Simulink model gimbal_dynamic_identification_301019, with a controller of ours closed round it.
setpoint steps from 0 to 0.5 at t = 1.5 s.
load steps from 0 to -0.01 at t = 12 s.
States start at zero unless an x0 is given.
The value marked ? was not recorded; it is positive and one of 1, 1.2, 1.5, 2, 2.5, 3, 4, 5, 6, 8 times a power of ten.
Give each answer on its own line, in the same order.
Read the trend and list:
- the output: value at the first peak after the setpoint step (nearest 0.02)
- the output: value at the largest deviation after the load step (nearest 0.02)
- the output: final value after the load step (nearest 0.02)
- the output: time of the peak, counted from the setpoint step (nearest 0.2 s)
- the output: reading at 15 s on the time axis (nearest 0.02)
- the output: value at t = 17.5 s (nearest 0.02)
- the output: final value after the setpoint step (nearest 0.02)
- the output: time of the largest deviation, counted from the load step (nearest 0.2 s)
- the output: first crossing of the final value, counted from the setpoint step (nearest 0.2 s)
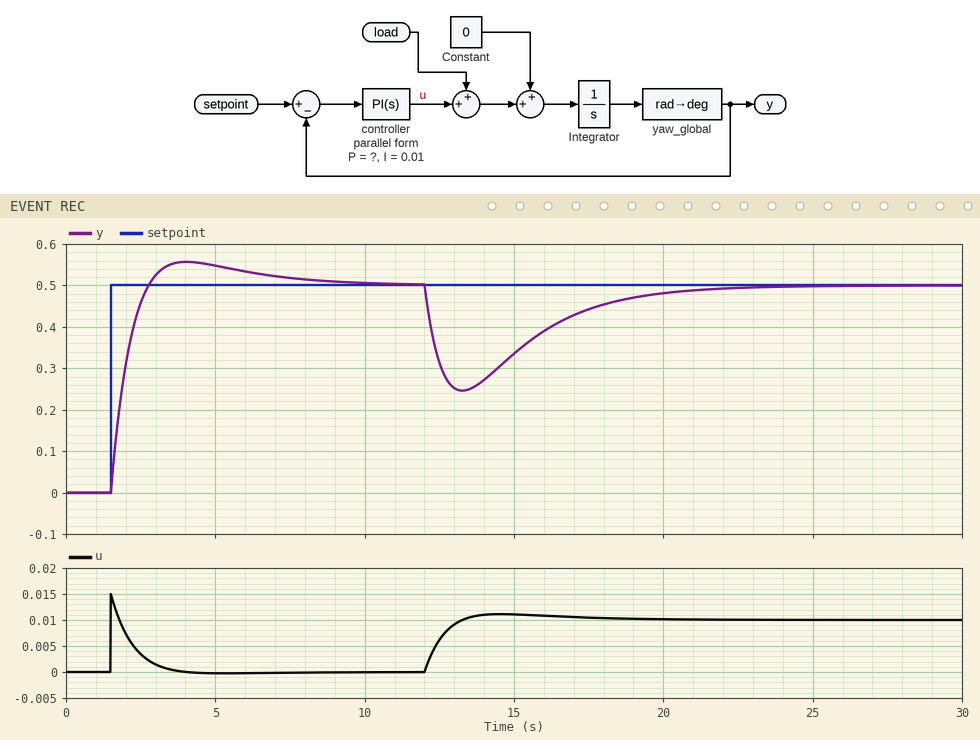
0.56
0.24
0.50
2.6 s
0.34
0.44
0.50
1.2 s
1.2 s
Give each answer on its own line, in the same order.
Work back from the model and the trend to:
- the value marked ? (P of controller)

0.03
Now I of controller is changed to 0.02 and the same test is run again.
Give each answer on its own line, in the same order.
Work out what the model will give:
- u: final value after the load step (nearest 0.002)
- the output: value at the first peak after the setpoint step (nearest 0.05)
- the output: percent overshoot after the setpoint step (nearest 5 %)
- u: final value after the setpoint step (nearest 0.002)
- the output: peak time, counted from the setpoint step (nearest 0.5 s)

0.010
0.60
20 %
0.000
2.0 s
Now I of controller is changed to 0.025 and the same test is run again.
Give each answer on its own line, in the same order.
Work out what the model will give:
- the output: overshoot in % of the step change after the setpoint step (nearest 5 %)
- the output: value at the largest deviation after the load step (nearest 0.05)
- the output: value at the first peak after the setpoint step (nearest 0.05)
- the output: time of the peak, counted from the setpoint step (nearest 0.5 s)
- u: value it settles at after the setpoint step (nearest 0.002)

20 %
0.30
0.60
2.0 s
0.000
